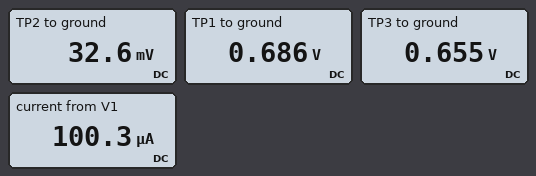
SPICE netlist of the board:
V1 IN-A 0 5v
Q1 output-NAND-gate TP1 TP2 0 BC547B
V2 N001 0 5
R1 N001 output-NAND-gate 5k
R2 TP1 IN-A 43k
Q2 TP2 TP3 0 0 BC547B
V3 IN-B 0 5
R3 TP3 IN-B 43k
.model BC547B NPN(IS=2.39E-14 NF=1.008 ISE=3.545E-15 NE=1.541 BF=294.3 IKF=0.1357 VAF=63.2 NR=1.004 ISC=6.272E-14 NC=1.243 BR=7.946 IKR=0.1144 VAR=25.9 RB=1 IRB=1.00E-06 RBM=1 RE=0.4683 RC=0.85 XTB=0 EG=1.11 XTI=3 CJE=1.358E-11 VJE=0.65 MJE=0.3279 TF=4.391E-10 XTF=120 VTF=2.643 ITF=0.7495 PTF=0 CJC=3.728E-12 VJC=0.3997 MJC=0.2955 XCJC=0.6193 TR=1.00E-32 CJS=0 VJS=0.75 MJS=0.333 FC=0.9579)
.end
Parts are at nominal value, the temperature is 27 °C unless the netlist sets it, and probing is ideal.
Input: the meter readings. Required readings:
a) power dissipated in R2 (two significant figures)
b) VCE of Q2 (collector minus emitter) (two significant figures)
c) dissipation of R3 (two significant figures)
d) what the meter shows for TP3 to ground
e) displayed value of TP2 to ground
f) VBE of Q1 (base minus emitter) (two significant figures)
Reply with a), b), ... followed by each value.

a) 430 µW
b) 33 mV
c) 440 µW
d) 0.655 V
e) 32.6 mV
f) 650 mV
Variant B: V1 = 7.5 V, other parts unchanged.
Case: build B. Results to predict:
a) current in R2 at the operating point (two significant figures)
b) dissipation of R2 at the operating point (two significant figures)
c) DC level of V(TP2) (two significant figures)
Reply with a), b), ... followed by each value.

a) 160 µA
b) 1.1 mW
c) 34 mV
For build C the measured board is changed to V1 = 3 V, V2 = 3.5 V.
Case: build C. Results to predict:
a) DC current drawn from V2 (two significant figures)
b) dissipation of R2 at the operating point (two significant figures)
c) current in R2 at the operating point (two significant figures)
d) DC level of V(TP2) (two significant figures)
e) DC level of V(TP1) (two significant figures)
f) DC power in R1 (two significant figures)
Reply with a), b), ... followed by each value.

a) 690 µA
b) 130 µW
c) 54 µA
d) 26 mV
e) 670 mV
f) 2.4 mW
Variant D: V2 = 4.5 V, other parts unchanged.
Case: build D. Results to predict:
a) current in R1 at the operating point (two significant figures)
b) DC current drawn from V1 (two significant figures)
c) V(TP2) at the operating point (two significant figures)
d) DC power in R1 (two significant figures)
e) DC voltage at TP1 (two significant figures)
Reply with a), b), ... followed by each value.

a) 890 µA
b) 100 µA
c) 31 mV
d) 3.9 mW
e) 680 mV
